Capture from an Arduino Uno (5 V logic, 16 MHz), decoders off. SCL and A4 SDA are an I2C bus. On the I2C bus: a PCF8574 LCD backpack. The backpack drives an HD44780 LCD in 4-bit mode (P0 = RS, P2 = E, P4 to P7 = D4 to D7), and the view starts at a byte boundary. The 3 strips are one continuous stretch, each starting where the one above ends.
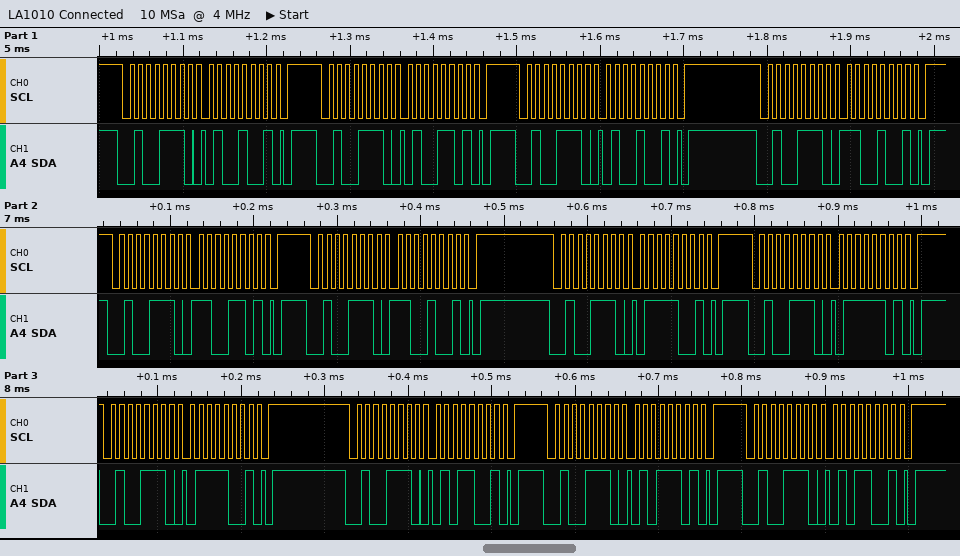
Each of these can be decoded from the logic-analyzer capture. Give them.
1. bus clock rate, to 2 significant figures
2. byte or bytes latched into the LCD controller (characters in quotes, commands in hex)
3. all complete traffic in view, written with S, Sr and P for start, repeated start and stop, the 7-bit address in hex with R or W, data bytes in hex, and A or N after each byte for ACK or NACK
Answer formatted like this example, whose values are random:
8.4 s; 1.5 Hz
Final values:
100 kHz; 'L' 'u'; S 27W A 49 A P S 27W A 4D A P S 27W A 49 A P S 27W A C9 A P S 27W A CD A P S 27W A C9 A P S 27W A 79 A P S 27W A 7D A P S 27W A 79 A P S 27W A 59 A P S 27W A 5D A P S 27W A 59 A P
